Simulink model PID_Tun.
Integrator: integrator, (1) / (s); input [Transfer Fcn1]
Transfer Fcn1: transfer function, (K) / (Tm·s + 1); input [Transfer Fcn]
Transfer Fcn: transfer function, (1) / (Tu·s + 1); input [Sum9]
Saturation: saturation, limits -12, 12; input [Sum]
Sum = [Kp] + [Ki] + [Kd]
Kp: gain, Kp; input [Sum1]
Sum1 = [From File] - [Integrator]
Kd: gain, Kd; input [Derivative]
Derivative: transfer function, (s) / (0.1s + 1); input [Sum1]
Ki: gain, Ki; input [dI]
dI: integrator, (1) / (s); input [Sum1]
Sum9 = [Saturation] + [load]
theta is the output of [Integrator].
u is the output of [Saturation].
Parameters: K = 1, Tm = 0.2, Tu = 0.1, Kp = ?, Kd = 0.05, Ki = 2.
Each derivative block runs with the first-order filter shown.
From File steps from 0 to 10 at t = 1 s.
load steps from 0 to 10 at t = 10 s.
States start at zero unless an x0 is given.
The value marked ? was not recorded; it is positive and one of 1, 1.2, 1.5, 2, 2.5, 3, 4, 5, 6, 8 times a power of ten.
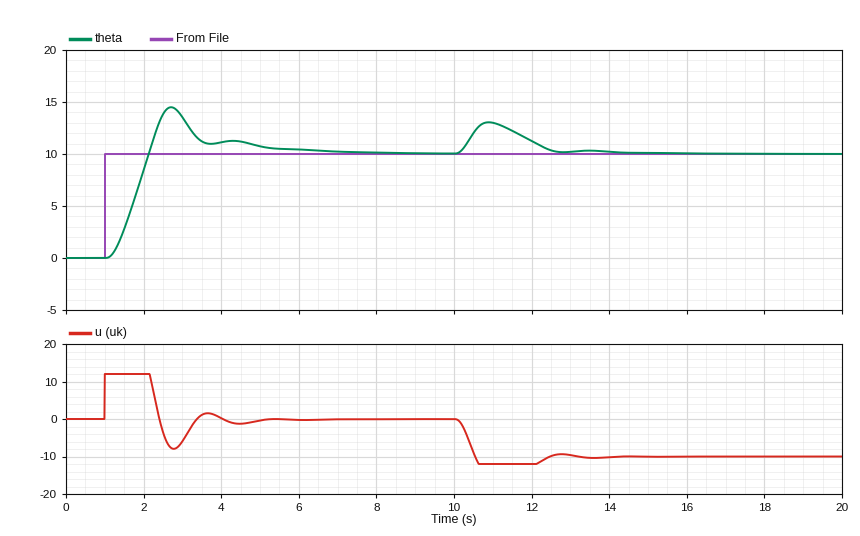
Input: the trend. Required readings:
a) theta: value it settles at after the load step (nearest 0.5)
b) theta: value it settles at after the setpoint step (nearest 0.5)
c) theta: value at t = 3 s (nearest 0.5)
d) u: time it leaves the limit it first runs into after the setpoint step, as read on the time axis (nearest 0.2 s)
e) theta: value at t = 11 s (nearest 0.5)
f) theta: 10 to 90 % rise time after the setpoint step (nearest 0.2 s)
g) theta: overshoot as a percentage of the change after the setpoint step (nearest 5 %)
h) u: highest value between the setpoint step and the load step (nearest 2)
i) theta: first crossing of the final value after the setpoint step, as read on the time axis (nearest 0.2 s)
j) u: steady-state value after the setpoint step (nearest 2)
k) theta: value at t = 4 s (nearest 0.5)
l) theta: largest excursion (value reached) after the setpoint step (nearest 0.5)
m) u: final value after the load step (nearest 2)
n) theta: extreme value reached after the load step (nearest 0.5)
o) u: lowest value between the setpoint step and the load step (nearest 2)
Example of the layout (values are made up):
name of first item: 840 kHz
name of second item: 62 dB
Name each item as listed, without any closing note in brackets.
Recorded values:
theta: value it settles at after the load step: 10.0
theta: value it settles at after the setpoint step: 10.0
theta: value at t = 3 s: 13.5
u: time it leaves the limit it first runs into after the setpoint step, as read on the time axis: 2.2 s
theta: value at t = 11 s: 13.0
theta: 10 to 90 % rise time after the setpoint step: 0.8 s
theta: overshoot as a percentage of the change after the setpoint step: 45 %
u: highest value between the setpoint step and the load step: 12
theta: first crossing of the final value after the setpoint step, as read on the time axis: 2.2 s
u: steady-state value after the setpoint step: 0
theta: value at t = 4 s: 11.0
theta: largest excursion (value reached) after the setpoint step: 14.5
u: final value after the load step: -10
theta: extreme value reached after the load step: 13.0
u: lowest value between the setpoint step and the load step: -8
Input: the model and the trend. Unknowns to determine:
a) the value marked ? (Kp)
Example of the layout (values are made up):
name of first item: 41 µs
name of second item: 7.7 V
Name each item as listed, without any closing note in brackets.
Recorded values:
the value marked ?: 4
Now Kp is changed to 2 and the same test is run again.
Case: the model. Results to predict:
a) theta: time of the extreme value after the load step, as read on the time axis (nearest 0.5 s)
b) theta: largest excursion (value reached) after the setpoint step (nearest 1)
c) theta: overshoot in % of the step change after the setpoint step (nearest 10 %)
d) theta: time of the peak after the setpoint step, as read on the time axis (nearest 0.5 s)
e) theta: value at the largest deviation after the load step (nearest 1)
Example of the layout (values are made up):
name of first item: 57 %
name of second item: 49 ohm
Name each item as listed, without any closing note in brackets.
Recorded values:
theta: time of the extreme value after the load step, as read on the time axis: 11.0 s
theta: largest excursion (value reached) after the setpoint step: 16
theta: overshoot in % of the step change after the setpoint step: 60 %
theta: time of the peak after the setpoint step, as read on the time axis: 3.0 s
theta: value at the largest deviation after the load step: 14
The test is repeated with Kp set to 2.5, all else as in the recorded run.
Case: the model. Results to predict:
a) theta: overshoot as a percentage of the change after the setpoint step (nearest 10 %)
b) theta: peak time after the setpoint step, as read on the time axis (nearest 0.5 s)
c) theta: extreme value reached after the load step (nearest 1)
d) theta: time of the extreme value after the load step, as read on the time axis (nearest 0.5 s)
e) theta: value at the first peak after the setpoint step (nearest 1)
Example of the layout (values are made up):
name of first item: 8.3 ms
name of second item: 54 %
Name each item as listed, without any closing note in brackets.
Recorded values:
theta: overshoot as a percentage of the change after the setpoint step: 60 %
theta: peak time after the setpoint step, as read on the time axis: 3.0 s
theta: extreme value reached after the load step: 14
theta: time of the extreme value after the load step, as read on the time axis: 11.0 s
theta: value at the first peak after the setpoint step: 16
